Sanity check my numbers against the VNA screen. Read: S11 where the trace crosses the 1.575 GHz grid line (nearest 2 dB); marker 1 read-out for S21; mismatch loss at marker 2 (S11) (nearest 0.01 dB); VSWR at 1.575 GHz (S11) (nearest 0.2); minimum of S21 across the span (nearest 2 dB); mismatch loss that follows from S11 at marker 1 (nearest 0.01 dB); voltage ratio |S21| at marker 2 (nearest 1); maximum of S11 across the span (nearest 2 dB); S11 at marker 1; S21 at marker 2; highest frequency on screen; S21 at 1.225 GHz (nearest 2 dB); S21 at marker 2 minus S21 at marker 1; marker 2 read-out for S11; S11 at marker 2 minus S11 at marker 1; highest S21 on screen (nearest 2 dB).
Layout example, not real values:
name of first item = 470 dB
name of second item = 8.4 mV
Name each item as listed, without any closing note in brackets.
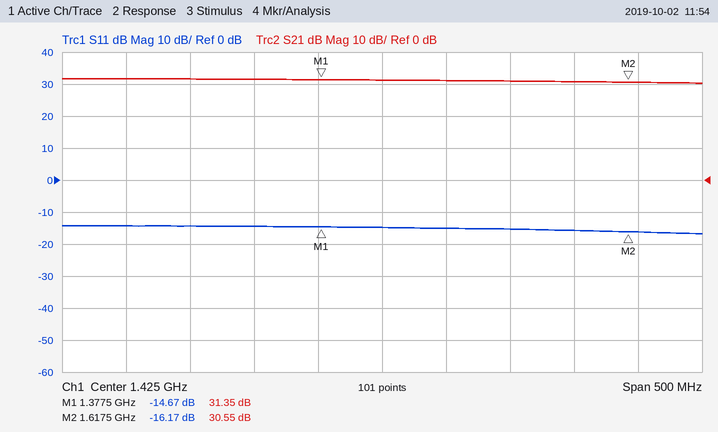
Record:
S11 where the trace crosses the 1.575 GHz grid line = -16 dB
marker 1 read-out for S21 = 31.35 dB
mismatch loss at marker 2 (S11) = 0.11 dB
VSWR at 1.575 GHz (S11) = 1.4
minimum of S21 across the span = 30 dB
mismatch loss that follows from S11 at marker 1 = 0.15 dB
voltage ratio |S21| at marker 2 = 34
maximum of S11 across the span = -14 dB
S11 at marker 1 = -14.67 dB
S21 at marker 2 = 30.55 dB
highest frequency on screen = 1.675 GHz
S21 at 1.225 GHz = 32 dB
S21 at marker 2 minus S21 at marker 1 = -0.80 dB
marker 2 read-out for S11 = -16.17 dB
S11 at marker 2 minus S11 at marker 1 = -1.50 dB
highest S21 on screen = 32 dB
